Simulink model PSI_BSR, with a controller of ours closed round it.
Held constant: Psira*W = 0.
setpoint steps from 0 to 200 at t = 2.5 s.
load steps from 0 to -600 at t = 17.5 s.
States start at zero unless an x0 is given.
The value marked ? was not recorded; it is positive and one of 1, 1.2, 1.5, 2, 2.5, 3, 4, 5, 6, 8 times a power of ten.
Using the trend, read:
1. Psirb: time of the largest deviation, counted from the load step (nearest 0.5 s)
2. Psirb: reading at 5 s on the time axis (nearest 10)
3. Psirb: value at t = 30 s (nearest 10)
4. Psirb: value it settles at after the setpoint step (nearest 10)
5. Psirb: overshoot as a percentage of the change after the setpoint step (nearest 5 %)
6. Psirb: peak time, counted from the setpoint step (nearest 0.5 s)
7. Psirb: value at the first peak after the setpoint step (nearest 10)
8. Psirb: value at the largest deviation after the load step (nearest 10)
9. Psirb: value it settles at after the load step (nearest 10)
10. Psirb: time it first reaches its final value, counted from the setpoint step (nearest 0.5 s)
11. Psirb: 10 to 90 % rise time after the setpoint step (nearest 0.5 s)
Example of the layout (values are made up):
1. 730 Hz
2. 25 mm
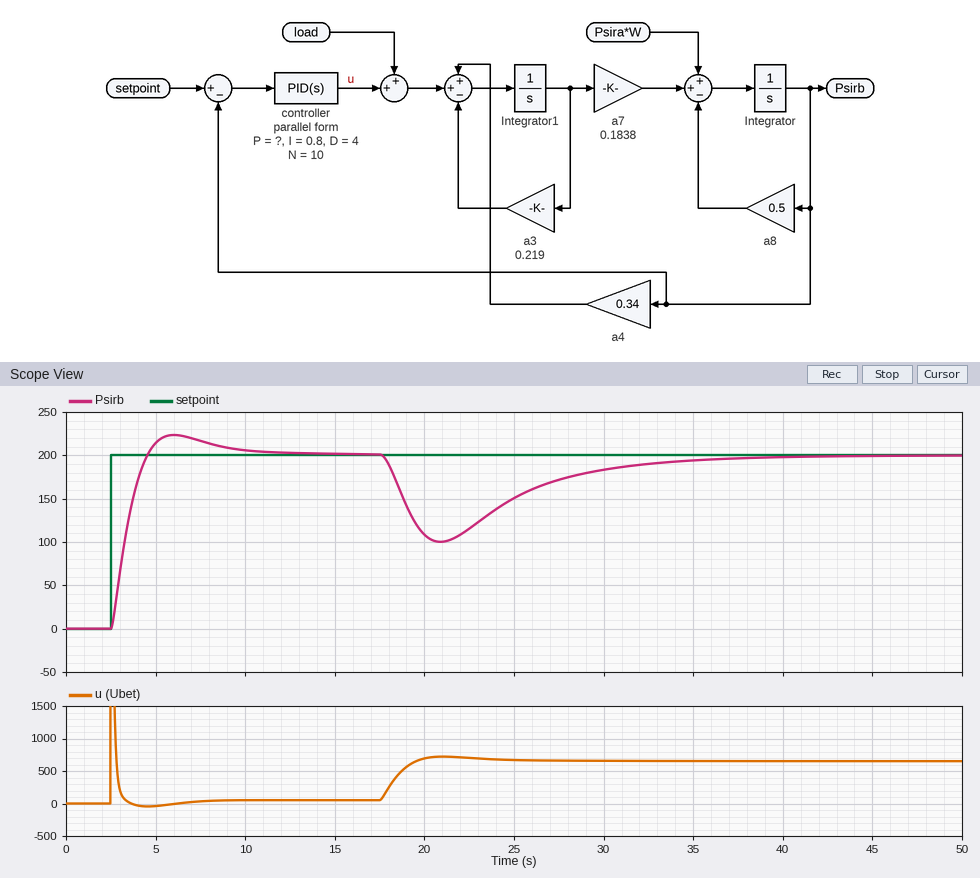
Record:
1. 3.5 s
2. 210
3. 180
4. 200
5. 10 %
6. 3.5 s
7. 220
8. 100
9. 200
10. 2.0 s
11. 1.5 s
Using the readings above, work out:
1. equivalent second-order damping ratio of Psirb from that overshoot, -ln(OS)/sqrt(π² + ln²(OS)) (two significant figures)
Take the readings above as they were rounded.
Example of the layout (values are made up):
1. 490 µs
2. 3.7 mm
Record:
1. 0.59
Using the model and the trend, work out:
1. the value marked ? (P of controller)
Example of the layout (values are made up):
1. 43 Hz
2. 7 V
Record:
1. 5
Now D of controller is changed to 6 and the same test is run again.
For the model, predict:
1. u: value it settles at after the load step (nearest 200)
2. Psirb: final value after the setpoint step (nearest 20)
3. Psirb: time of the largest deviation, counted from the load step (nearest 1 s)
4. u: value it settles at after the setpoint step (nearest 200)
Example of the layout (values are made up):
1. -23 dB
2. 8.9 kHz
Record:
1. 600
2. 200
3. 4 s
4. 0
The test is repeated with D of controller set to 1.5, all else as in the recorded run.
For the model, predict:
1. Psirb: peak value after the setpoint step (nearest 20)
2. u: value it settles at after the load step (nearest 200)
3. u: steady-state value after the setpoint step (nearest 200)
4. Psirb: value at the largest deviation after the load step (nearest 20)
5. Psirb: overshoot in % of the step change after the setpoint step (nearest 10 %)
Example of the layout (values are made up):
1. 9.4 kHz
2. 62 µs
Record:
1. 260
2. 600
3. 0
4. 80
5. 30 %
